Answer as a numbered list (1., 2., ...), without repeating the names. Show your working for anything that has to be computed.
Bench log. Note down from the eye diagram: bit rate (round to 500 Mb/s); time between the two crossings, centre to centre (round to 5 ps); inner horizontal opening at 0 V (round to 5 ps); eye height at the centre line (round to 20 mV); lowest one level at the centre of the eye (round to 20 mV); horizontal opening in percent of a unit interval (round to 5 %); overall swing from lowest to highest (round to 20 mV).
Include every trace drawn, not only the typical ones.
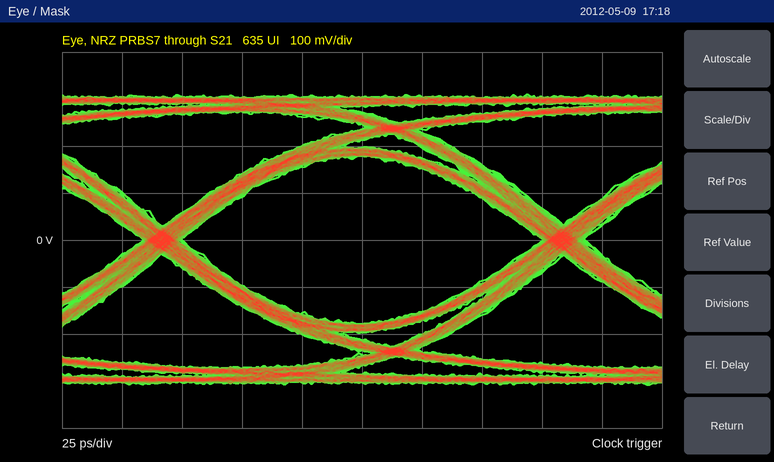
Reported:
1. 6.0 Gb/s
2. 165 ps
3. 150 ps
4. 360 mV
5. 180 mV
6. 150 ps / 165 ps ≈ 90.9 %, so 90 % to the nearest 5 %
7. 620 mV
